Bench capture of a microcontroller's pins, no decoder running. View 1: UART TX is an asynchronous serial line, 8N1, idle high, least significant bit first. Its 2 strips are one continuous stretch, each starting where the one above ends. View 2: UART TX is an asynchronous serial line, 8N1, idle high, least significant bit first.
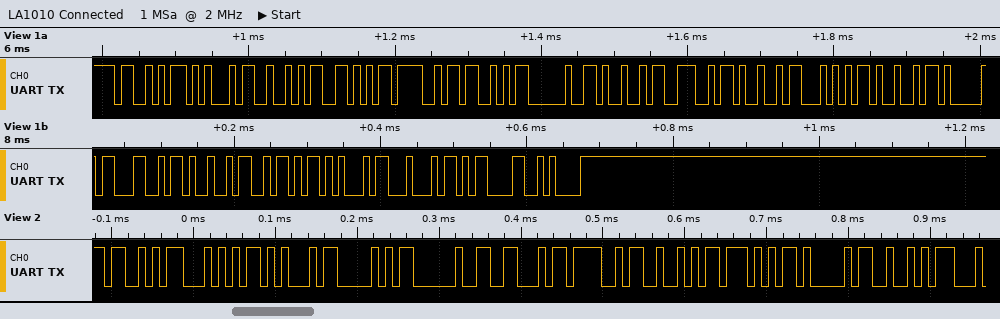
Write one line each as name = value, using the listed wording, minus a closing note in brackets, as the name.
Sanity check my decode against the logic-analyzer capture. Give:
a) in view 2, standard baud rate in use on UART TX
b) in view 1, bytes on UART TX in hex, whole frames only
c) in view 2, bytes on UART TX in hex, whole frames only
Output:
in view 2, standard baud rate in use on UART TX = 115200 baud
in view 1, bytes on UART TX in hex, whole frames only = 53 45 52 56 4F 53 20 49 4E 49 54 49 41 4C 49 5A 45 44 0D 0A
in view 2, bytes on UART TX in hex, whole frames only = 53 54 45 50 20 46 4F 52 57 41 52
